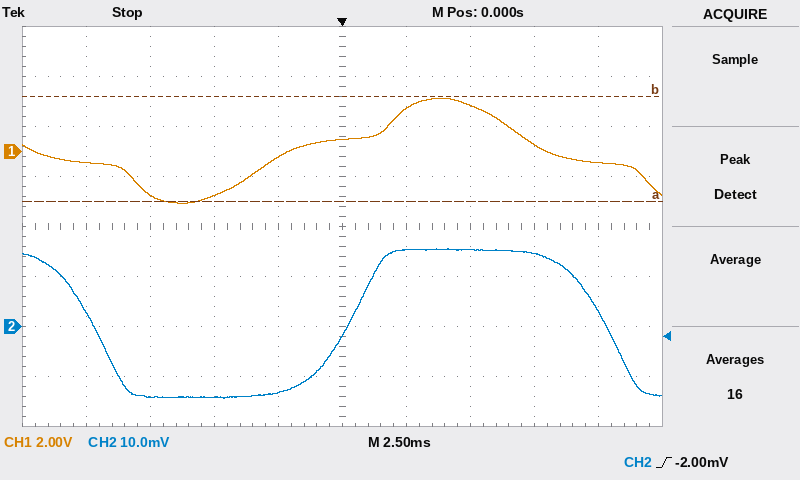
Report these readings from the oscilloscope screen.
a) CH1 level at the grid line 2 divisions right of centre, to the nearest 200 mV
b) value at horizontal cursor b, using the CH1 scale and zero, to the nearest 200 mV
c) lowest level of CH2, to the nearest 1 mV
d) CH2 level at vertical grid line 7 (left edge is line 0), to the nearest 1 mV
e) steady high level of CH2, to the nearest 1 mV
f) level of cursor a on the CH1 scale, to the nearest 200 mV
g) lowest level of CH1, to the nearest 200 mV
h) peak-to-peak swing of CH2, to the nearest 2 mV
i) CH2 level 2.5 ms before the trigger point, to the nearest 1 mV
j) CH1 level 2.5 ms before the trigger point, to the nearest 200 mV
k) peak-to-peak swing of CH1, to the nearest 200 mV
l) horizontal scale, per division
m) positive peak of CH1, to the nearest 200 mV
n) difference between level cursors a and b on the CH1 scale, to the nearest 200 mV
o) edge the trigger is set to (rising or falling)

1.8 V
2.2 V
-14 mV
15 mV
15 mV
-2.0 V
-2.0 V
30 mV
-13 mV
-200 mV
4.2 V
2.5 ms
2.2 V
4.2 V
rising
